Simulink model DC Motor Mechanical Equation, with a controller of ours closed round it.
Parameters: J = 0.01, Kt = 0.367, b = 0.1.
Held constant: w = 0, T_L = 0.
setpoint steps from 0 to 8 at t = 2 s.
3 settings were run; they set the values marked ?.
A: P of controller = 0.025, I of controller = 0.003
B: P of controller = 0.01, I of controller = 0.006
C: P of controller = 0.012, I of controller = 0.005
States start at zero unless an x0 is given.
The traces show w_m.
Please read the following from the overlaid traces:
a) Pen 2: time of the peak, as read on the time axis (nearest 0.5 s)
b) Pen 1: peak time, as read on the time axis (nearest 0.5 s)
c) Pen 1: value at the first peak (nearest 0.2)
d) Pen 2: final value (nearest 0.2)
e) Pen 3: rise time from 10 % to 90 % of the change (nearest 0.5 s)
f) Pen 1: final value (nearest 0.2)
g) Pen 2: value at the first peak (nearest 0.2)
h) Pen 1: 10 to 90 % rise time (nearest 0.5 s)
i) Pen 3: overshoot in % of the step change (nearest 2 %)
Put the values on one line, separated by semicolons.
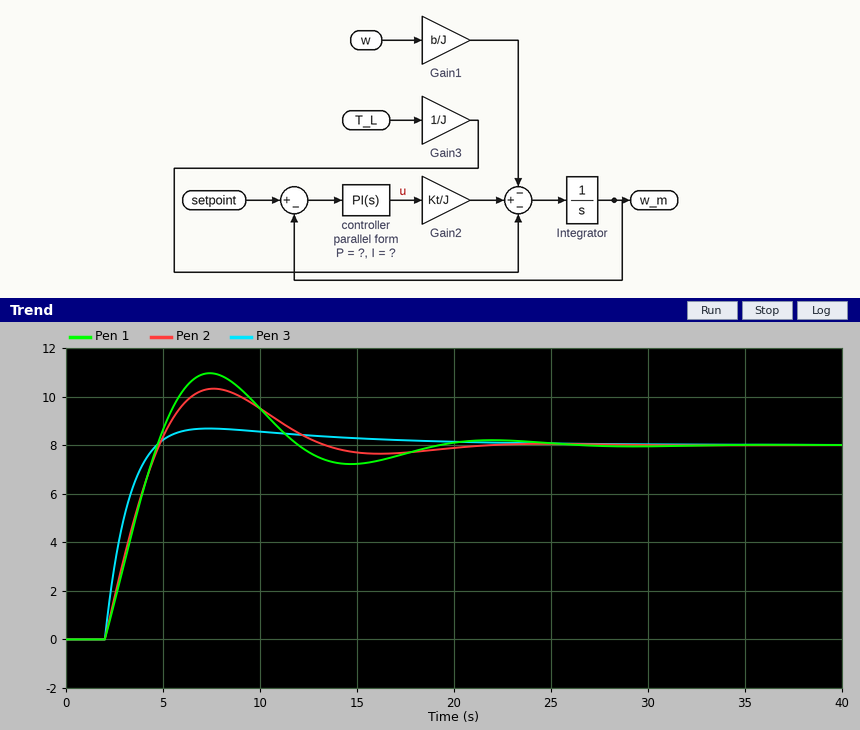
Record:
7.5 s; 7.5 s; 11.0; 8.0; 2.0 s; 8.0; 10.4; 2.0 s; 8 %
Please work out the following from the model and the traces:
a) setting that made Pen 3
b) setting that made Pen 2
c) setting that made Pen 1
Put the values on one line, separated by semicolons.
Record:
A; C; B
